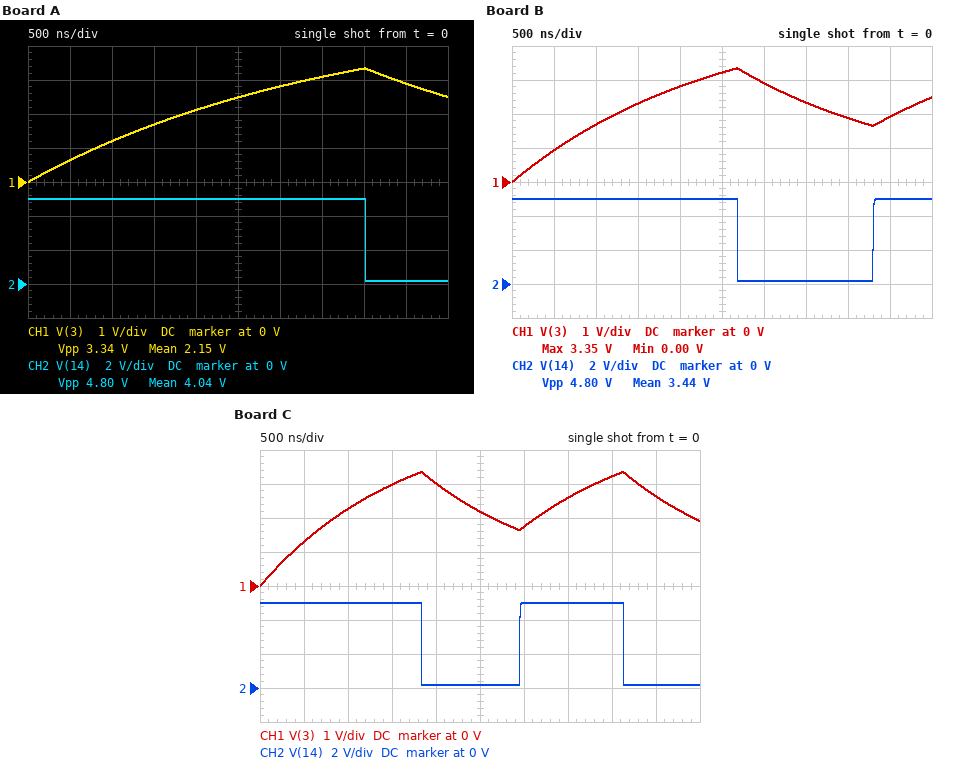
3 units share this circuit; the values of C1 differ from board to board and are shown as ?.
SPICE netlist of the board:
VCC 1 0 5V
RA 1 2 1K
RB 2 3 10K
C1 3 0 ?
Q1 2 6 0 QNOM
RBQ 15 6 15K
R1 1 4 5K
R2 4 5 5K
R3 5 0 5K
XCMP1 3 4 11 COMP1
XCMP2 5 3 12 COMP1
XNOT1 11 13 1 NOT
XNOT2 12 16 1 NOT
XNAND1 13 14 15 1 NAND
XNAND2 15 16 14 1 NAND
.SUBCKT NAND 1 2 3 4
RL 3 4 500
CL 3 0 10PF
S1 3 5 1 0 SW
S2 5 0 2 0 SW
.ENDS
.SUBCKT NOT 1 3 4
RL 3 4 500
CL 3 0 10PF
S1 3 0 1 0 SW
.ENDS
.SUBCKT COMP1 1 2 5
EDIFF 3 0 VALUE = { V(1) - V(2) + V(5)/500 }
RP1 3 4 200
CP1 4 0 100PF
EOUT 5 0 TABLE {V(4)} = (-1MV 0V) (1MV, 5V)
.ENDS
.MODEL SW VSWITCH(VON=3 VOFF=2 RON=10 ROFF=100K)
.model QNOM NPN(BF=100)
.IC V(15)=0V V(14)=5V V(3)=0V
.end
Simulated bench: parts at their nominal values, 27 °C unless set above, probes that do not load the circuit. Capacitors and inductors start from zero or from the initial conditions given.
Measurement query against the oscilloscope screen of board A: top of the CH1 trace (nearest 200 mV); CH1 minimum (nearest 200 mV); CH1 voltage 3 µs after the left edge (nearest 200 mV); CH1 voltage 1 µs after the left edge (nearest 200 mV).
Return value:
3.4 V
0 V
2.8 V
1.2 V
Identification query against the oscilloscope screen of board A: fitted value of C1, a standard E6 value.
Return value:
330 pF
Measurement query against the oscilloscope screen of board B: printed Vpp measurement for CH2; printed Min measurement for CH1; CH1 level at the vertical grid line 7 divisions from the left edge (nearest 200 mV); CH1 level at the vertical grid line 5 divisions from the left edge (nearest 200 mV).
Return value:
4.80 V
0.00 V
2.4 V
3.2 V
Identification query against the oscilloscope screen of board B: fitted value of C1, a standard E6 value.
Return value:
220 pF
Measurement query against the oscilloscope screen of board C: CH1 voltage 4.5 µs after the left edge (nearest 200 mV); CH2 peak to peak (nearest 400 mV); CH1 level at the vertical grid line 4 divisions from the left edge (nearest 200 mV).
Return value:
2.6 V
4.8 V
3.0 V
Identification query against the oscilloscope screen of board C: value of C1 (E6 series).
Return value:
150 pF
